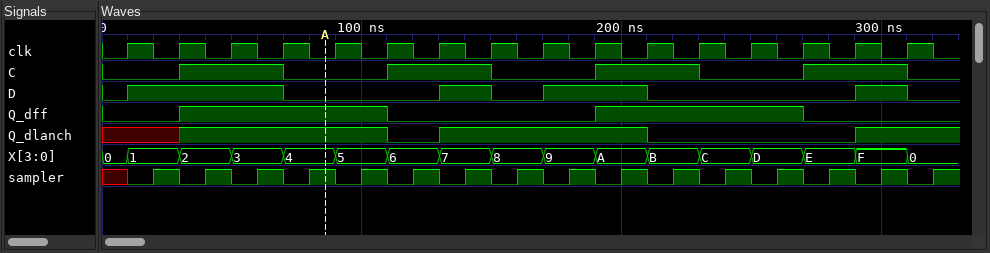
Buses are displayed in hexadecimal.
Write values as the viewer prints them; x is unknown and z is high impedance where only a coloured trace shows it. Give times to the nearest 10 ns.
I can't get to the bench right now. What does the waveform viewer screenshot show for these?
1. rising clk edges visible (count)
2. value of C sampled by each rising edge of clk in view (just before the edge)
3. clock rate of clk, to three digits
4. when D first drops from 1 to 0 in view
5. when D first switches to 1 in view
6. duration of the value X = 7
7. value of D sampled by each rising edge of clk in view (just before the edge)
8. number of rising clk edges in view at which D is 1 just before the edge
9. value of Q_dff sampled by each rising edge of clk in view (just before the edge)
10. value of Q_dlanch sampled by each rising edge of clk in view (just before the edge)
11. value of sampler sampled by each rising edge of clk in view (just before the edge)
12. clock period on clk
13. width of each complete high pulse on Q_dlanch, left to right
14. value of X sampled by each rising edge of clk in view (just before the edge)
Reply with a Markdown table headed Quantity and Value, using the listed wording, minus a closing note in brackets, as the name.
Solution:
| Quantity | Value |
|---|---|
| rising clk edges visible | 16 |
| value of C sampled by each rising edge of clk in view | 0 0 1 1 0 0 1 1 0 0 1 1 0 0 1 1 |
| clock rate of clk, to three digits | 50.0 MHz |
| when D first drops from 1 to 0 in view | 70 ns |
| when D first switches to 1 in view | 10 ns |
| duration of the value X = 7 | 20 ns |
| value of D sampled by each rising edge of clk in view | 0 1 1 1 0 0 0 1 0 1 1 0 0 0 0 1 |
| number of rising clk edges in view at which D is 1 just before the edge | 7 |
| value of Q_dff sampled by each rising edge of clk in view | 0 0 1 1 1 1 0 0 0 0 1 1 1 1 0 0 |
| value of Q_dlanch sampled by each rising edge of clk in view | x x 1 1 1 1 0 1 1 1 1 0 0 0 0 1 |
| value of sampler sampled by each rising edge of clk in view | x 1 1 1 1 1 1 1 1 1 1 1 1 1 1 1 |
| clock period on clk | 20 ns |
| width of each complete high pulse on Q_dlanch, left to right | 80 ns |
| value of X sampled by each rising edge of clk in view | 0, 1, 2, 3, 4, 5, 6, 7, 8, 9, A, B, C, D, E, F |
